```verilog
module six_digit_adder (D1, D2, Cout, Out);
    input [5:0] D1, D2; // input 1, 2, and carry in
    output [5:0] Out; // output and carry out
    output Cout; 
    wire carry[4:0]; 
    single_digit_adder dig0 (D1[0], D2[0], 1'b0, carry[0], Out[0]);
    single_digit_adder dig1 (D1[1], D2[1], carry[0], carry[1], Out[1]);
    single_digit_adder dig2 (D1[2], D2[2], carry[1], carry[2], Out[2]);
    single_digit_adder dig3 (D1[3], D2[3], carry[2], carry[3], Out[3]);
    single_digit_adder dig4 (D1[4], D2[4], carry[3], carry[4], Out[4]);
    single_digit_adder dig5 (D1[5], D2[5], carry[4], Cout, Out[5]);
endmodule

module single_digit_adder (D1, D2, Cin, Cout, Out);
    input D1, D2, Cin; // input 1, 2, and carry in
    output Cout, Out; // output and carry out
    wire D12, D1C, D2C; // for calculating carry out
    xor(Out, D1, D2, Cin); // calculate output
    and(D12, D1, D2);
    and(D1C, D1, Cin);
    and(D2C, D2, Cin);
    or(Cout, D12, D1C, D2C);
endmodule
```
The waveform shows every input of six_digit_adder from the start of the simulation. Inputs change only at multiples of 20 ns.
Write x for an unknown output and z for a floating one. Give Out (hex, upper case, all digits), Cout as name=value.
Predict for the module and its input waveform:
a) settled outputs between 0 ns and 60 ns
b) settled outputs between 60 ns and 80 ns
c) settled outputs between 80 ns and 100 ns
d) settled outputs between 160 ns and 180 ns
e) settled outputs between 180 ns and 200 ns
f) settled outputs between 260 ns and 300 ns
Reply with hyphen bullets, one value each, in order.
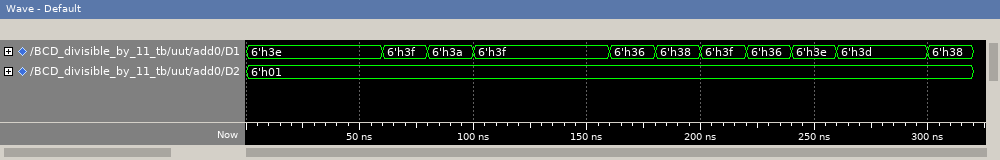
- Out=3F, Cout=0
- Out=00, Cout=1
- Out=3B, Cout=0
- Out=37, Cout=0
- Out=39, Cout=0
- Out=3E, Cout=0
